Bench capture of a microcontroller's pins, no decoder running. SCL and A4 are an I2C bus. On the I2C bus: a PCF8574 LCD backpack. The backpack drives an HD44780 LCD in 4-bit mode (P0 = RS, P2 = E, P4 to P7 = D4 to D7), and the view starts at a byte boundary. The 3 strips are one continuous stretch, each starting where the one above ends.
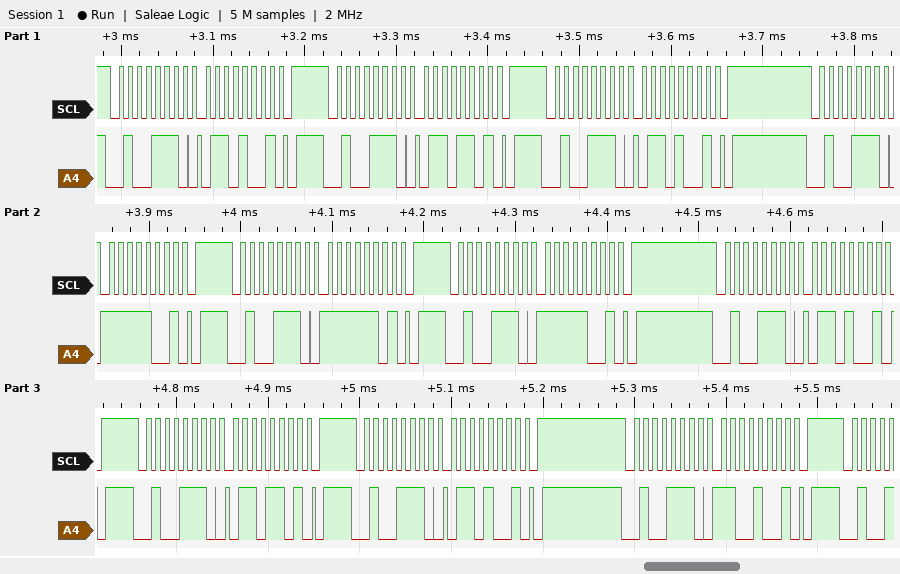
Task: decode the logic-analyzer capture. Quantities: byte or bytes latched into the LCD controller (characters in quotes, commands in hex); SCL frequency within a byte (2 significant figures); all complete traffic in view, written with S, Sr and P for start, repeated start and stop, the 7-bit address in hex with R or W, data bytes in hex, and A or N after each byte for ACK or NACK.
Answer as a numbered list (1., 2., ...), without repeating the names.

1. 'o'
2. 100 kHz
3. S 27W A 69 A P S 27W A 6D A P S 27W A 69 A P S 27W A F9 A P S 27W A FD A P S 27W A F9 A P S 27W A 69 A P S 27W A 6D A P S 27W A 69 A P S 27W A C9 A P
